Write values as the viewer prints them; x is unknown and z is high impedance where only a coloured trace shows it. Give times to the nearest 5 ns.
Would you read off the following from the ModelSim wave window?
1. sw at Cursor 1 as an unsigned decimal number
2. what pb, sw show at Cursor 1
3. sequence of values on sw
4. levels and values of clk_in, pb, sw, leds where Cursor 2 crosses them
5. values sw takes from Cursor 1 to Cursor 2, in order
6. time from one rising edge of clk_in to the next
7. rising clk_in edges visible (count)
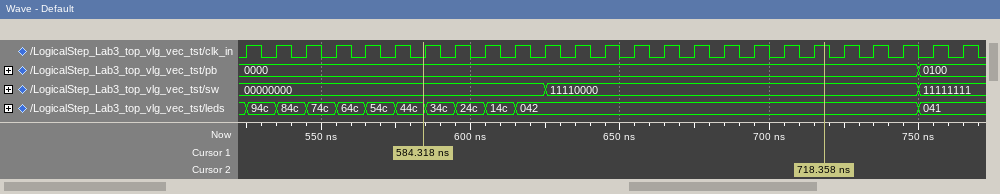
0
pb=0000, sw=00000000
00000000, 11110000, 11111111
clk_in=1, pb=0000, sw=11110000, leds=042
00000000, 11110000
10 ns
25
